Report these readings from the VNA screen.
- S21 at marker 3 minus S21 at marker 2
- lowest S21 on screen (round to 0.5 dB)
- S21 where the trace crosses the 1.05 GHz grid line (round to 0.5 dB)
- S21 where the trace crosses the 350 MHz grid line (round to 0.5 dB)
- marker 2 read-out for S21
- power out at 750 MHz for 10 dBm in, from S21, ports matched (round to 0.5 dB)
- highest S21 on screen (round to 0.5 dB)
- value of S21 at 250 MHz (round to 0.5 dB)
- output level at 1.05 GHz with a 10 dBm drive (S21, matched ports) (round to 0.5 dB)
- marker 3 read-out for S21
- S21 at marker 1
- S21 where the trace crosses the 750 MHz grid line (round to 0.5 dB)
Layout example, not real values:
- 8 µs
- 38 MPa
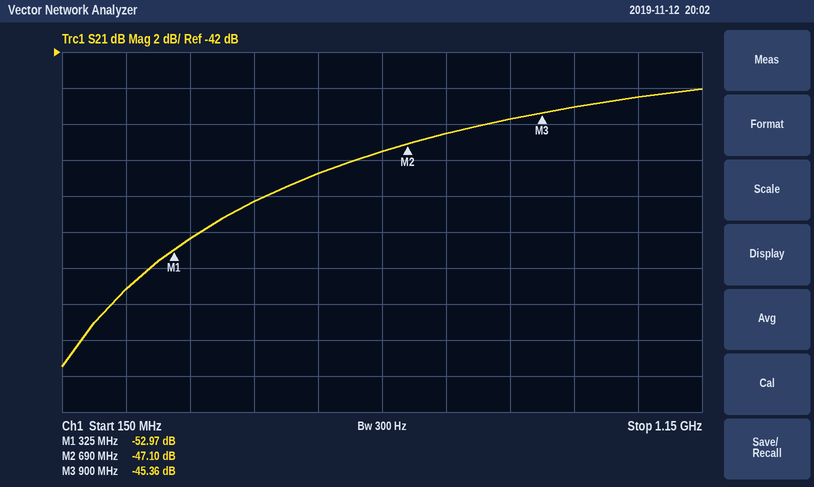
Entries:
- 1.74 dB
- -59.5 dB
- -44.5 dB
- -52.5 dB
- -47.10 dB
- -36.5 dBm
- -44.0 dB
- -55.0 dB
- -34.5 dBm
- -45.36 dB
- -52.97 dB
- -46.5 dB
